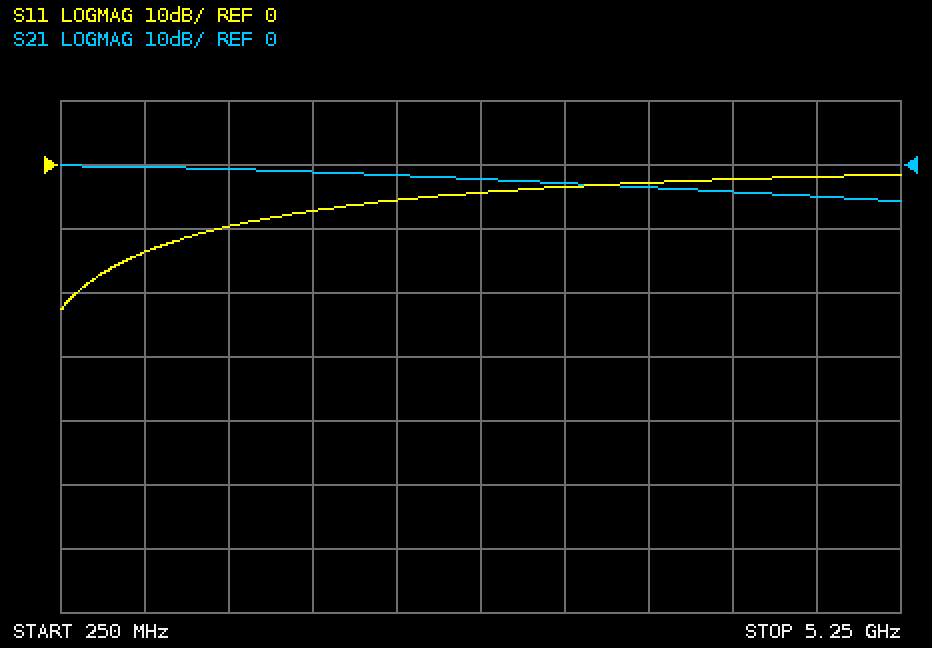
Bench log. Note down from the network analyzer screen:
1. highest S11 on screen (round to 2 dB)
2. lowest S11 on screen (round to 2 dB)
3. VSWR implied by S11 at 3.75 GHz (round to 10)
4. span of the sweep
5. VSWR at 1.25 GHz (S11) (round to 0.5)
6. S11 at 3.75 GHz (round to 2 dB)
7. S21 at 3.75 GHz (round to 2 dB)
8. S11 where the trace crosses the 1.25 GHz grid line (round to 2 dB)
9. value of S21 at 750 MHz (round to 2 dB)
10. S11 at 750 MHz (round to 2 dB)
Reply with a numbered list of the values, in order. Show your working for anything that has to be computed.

1. -2 dB
2. -22 dB
3. |Γ| = 10^(-2/20) = 0.7943; VSWR = (1 + 0.7943)/(1 − 0.7943) ≈ 8.72, so 10 to the nearest 10
4. 5 GHz
5. |Γ| = 10^(-10/20) = 0.3162; VSWR = (1 + 0.3162)/(1 − 0.3162) ≈ 1.92, so 2.0 to the nearest 0.5
6. -2 dB
7. -4 dB
8. -10 dB
9. 0 dB
10. -14 dB
